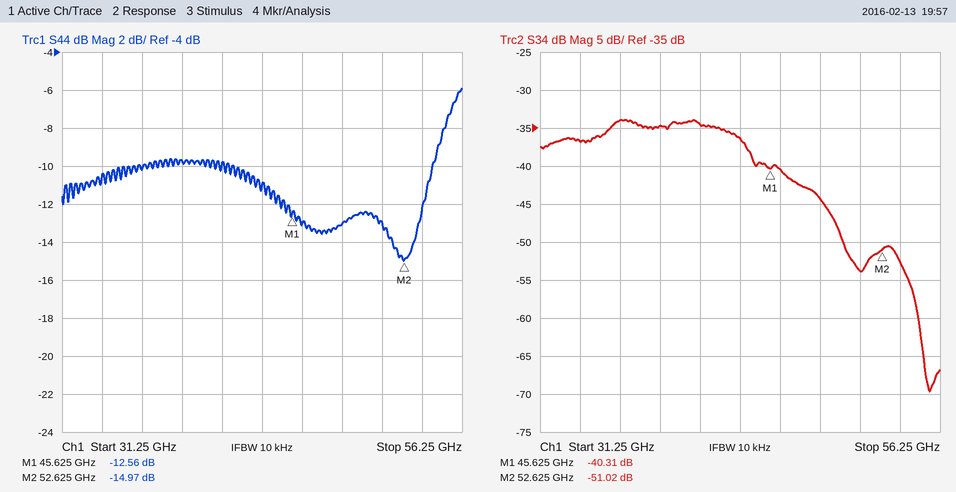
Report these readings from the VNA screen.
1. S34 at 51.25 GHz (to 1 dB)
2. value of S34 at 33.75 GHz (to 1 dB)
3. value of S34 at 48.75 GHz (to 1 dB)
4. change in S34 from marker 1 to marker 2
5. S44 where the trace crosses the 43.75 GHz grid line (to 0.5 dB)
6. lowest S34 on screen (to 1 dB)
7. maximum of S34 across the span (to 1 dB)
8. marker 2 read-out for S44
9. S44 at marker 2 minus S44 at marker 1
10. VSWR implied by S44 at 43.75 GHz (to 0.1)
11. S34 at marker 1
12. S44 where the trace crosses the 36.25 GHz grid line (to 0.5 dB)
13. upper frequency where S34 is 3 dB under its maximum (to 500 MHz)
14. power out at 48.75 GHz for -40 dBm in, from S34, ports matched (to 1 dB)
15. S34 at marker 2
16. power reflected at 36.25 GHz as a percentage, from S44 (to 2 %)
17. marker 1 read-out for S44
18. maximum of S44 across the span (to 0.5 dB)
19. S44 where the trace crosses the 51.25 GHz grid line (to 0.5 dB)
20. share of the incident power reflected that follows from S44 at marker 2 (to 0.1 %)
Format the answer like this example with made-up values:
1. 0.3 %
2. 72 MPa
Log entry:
1. -54 dB
2. -37 dB
3. -44 dB
4. -10.71 dB
5. -11.0 dB
6. -70 dB
7. -34 dB
8. -14.97 dB
9. -2.41 dB
10. 1.8
11. -40.31 dB
12. -10.0 dB
13. 44.0 GHz
14. -84 dBm
15. -51.02 dB
16. 10 %
17. -12.56 dB
18. -6.0 dB
19. -13.0 dB
20. 3.2 %
